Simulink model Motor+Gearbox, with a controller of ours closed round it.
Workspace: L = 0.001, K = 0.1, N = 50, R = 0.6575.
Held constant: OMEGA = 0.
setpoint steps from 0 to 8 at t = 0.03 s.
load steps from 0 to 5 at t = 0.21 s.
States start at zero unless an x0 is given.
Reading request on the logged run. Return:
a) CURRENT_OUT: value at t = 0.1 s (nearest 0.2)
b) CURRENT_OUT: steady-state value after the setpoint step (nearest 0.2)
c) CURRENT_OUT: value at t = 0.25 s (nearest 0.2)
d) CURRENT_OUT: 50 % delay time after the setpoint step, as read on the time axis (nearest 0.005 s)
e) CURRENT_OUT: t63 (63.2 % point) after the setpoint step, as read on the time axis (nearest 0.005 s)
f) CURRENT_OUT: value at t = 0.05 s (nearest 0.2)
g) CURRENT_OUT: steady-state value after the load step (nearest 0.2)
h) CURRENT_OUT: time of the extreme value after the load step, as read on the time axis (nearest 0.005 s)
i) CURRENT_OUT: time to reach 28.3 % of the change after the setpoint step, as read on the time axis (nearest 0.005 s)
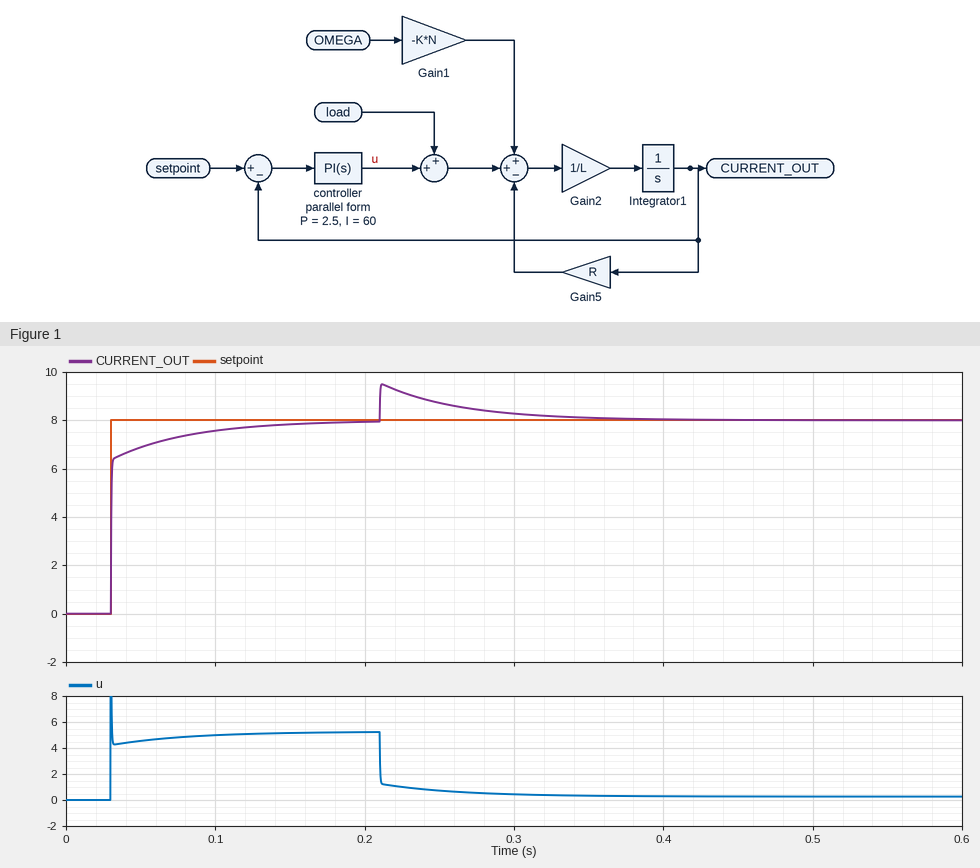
7.6
8.0
8.8
0.030 s
0.030 s
6.8
8.0
0.210 s
0.030 s
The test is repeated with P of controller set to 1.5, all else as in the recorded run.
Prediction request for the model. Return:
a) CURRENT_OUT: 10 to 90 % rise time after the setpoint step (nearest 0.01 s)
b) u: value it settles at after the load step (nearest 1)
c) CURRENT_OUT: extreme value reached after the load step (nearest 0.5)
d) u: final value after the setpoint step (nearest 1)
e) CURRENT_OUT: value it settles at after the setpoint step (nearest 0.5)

0.04 s
0
10.0
5
8.0
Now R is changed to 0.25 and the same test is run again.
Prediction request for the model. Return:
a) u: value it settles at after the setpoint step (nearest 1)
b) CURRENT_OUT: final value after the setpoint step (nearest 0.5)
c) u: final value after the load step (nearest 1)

2
8.0
-3
